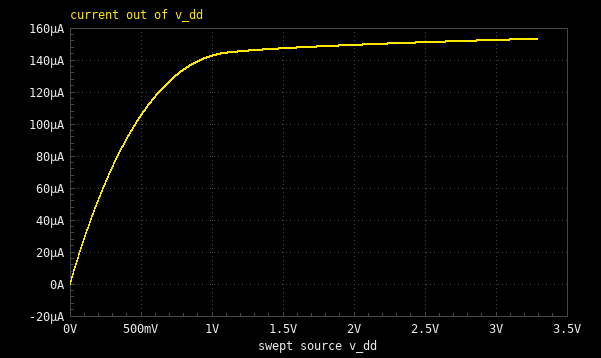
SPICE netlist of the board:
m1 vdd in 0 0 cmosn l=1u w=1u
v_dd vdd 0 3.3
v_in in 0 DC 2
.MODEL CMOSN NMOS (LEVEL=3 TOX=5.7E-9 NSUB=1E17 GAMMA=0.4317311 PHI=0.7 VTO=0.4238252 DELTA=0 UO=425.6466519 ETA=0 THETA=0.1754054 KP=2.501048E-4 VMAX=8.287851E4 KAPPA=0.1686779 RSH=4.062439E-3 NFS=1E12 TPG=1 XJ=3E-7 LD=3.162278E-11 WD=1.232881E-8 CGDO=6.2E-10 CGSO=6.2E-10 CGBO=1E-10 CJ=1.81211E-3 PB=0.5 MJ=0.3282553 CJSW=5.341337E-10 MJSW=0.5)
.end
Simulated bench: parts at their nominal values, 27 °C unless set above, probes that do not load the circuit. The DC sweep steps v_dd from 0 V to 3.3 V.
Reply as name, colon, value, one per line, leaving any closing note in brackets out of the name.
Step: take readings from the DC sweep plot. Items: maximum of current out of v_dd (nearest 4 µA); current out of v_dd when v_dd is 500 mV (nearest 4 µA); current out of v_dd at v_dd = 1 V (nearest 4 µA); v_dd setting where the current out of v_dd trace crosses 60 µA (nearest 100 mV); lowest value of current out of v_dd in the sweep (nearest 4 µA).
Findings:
maximum of current out of v_dd: 152 µA
current out of v_dd when v_dd is 500 mV: 104 µA
current out of v_dd at v_dd = 1 V: 144 µA
v_dd setting where the current out of v_dd trace crosses 60 µA: 200 mV
lowest value of current out of v_dd in the sweep: 0 A
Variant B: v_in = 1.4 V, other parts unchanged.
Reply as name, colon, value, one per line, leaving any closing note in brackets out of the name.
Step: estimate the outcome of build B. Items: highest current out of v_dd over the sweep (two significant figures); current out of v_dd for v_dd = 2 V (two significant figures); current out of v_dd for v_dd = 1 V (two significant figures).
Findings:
highest current out of v_dd over the sweep: 74 µA
current out of v_dd for v_dd = 2 V: 72 µA
current out of v_dd for v_dd = 1 V: 70 µA
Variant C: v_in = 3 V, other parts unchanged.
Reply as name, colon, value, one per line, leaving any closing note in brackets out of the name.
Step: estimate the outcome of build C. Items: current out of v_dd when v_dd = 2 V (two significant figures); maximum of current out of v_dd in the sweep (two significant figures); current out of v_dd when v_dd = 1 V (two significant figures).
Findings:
current out of v_dd when v_dd = 2 V: 300 µA
maximum of current out of v_dd in the sweep: 310 µA
current out of v_dd when v_dd = 1 V: 250 µA
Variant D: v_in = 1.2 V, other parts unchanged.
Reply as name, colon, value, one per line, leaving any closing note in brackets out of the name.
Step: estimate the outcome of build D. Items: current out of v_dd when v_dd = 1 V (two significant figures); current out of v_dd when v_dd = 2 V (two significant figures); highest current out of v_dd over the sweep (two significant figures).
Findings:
current out of v_dd when v_dd = 1 V: 49 µA
current out of v_dd when v_dd = 2 V: 50 µA
highest current out of v_dd over the sweep: 51 µA
